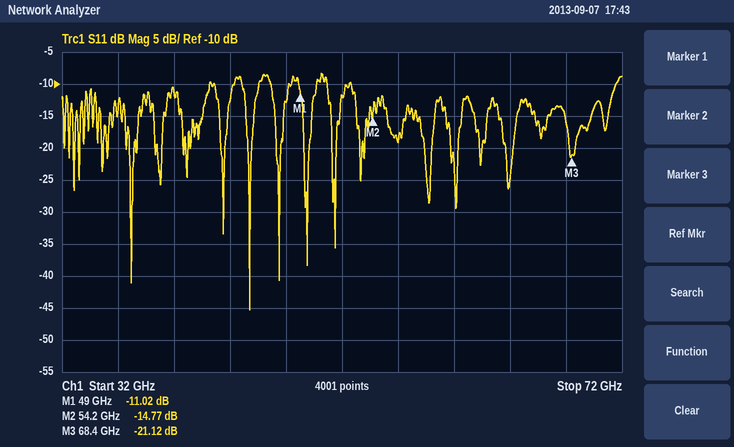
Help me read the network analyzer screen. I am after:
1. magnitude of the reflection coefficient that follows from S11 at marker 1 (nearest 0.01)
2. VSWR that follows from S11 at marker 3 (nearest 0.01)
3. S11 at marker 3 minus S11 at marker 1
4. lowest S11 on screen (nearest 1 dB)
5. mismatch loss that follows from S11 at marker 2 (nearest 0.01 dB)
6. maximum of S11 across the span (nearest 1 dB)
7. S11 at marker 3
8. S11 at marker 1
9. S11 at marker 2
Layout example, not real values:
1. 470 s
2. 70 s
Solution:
1. 0.28
2. 1.19
3. -10.10 dB
4. -45 dB
5. 0.15 dB
6. -8 dB
7. -21.12 dB
8. -11.02 dB
9. -14.77 dB
